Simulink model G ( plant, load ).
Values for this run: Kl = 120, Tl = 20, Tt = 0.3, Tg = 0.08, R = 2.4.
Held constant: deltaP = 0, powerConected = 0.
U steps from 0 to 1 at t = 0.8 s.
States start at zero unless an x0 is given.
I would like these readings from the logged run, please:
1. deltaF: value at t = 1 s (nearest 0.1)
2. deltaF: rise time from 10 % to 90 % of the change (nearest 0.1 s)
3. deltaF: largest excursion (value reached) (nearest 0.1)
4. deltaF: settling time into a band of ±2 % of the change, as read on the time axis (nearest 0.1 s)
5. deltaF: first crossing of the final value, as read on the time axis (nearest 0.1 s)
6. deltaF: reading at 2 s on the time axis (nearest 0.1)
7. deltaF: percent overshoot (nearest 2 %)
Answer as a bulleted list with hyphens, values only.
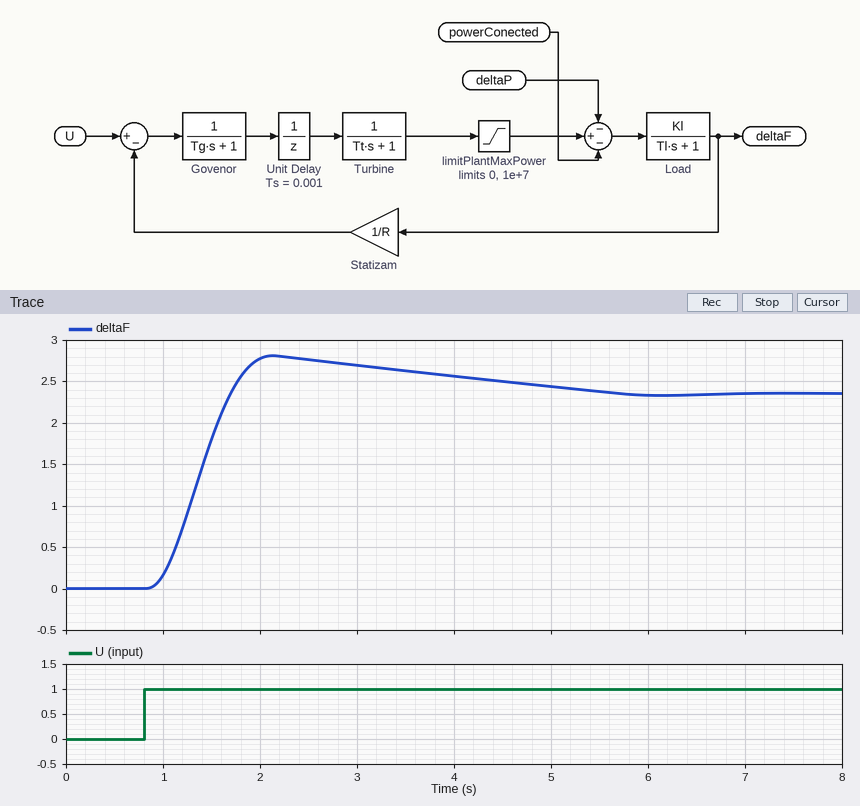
- 0.2
- 0.6 s
- 2.8
- 5.3 s
- 1.7 s
- 2.8
- 20 %
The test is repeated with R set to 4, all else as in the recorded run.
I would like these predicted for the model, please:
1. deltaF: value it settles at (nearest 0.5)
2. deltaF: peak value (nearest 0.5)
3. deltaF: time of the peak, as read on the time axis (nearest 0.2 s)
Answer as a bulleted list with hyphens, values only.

- 4.0
- 4.0
- 2.8 s
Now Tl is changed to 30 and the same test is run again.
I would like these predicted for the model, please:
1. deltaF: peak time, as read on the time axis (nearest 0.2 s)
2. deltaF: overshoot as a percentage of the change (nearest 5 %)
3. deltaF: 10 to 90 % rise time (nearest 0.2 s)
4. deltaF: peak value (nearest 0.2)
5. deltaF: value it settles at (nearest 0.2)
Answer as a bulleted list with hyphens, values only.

- 2.6 s
- 10 %
- 0.8 s
- 2.6
- 2.4
